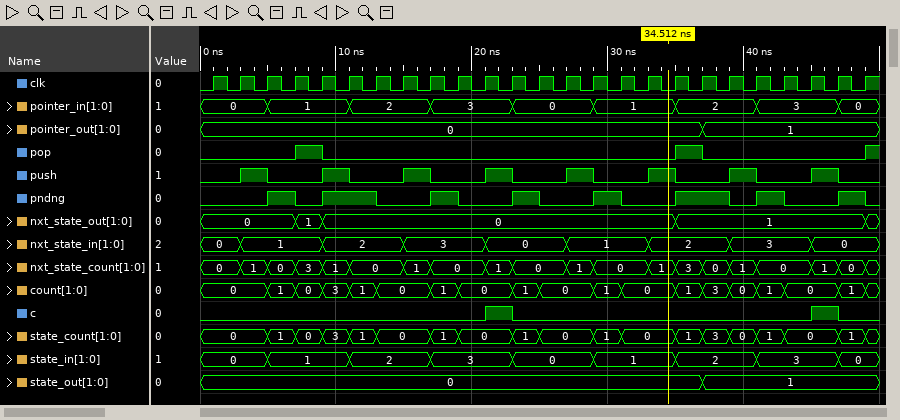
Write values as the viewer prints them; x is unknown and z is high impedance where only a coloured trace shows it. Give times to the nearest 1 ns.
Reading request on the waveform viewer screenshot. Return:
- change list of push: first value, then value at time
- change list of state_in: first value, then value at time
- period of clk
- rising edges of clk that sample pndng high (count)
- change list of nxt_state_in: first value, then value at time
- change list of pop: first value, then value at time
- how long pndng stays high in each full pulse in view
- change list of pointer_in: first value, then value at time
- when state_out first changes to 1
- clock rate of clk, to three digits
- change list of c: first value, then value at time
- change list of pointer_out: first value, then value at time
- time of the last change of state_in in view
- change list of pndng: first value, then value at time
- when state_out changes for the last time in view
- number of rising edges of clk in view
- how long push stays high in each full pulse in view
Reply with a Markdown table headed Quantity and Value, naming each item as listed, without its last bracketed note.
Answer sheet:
| Quantity | Value |
|---|---|
| change list of push: first value, then value at time | 0, 1 at 3 ns, 0 at 5 ns, 1 at 9 ns, 0 at 11 ns, 1 at 15 ns, 0 at 17 ns, 1 at 21 ns, 0 at 23 ns, 1 at 27 ns, 0 at 29 ns, 1 at 33 ns, 0 at 35 ns, 1 at 39 ns, 0 at 41 ns, 1 at 45 ns, 0 at 47 ns |
| change list of state_in: first value, then value at time | 0, 1 at 5 ns, 2 at 11 ns, 3 at 17 ns, 0 at 23 ns, 1 at 29 ns, 2 at 35 ns, 3 at 41 ns, 0 at 47 ns |
| period of clk | 2 ns |
| rising edges of clk that sample pndng high | 10 |
| change list of nxt_state_in: first value, then value at time | 0, 1 at 3 ns, 2 at 9 ns, 3 at 15 ns, 0 at 21 ns, 1 at 27 ns, 2 at 33 ns, 3 at 39 ns, 0 at 45 ns |
| change list of pop: first value, then value at time | 0, 1 at 7 ns, 0 at 9 ns, 1 at 35 ns, 0 at 37 ns, 1 at 49 ns |
| how long pndng stays high in each full pulse in view | 2 ns, 4 ns, 2 ns, 2 ns, 2 ns, 4 ns, 2 ns, 2 ns |
| change list of pointer_in: first value, then value at time | 0, 1 at 5 ns, 2 at 11 ns, 3 at 17 ns, 0 at 23 ns, 1 at 29 ns, 2 at 35 ns, 3 at 41 ns, 0 at 47 ns |
| when state_out first changes to 1 | 37 ns |
| clock rate of clk, to three digits | 500 MHz |
| change list of c: first value, then value at time | 0, 1 at 21 ns, 0 at 23 ns, 1 at 45 ns, 0 at 47 ns |
| change list of pointer_out: first value, then value at time | 0, 1 at 37 ns |
| time of the last change of state_in in view | 47 ns |
| change list of pndng: first value, then value at time | 0, 1 at 5 ns, 0 at 7 ns, 1 at 9 ns, 0 at 13 ns, 1 at 17 ns, 0 at 19 ns, 1 at 23 ns, 0 at 25 ns, 1 at 29 ns, 0 at 31 ns, 1 at 35 ns, 0 at 39 ns, 1 at 41 ns, 0 at 43 ns, 1 at 47 ns, 0 at 49 ns |
| when state_out changes for the last time in view | 37 ns |
| number of rising edges of clk in view | 25 |
| how long push stays high in each full pulse in view | 2 ns, 2 ns, 2 ns, 2 ns, 2 ns, 2 ns, 2 ns, 2 ns |
